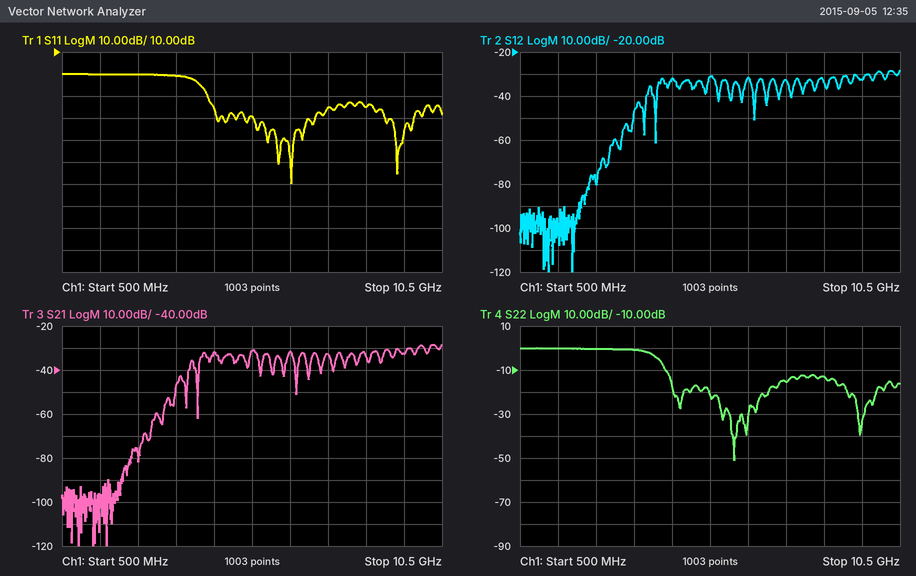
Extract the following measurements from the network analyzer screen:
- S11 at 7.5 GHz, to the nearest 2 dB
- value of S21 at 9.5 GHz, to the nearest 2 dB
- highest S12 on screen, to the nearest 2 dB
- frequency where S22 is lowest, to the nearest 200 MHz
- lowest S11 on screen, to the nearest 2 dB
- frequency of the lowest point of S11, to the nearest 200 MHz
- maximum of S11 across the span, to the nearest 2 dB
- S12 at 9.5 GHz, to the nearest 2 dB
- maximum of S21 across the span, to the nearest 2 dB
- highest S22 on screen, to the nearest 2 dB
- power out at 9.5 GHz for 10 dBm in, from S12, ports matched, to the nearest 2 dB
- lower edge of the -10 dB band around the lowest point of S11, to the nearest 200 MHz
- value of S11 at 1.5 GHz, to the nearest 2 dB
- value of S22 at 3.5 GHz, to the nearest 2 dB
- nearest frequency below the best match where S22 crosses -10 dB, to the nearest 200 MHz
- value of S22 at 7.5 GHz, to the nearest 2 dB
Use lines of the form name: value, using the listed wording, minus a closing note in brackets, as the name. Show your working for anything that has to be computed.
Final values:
S11 at 7.5 GHz, to the nearest 2 dB: -16 dB
value of S21 at 9.5 GHz, to the nearest 2 dB: -32 dB
highest S12 on screen, to the nearest 2 dB: -28 dB
frequency where S22 is lowest, to the nearest 200 MHz: 6.2 GHz
lowest S11 on screen, to the nearest 2 dB: -50 dB
frequency of the lowest point of S11, to the nearest 200 MHz: 6.6 GHz
maximum of S11 across the span, to the nearest 2 dB: 0 dB
S12 at 9.5 GHz, to the nearest 2 dB: -32 dB
maximum of S21 across the span, to the nearest 2 dB: -28 dB
highest S22 on screen, to the nearest 2 dB: 0 dB
power out at 9.5 GHz for 10 dBm in, from S12, ports matched, to the nearest 2 dB: 10 dBm + (-32 dB) = -22 dBm
lower edge of the -10 dB band around the lowest point of S11, to the nearest 200 MHz: 4.4 GHz
value of S11 at 1.5 GHz, to the nearest 2 dB: 0 dB
value of S22 at 3.5 GHz, to the nearest 2 dB: 0 dB
nearest frequency below the best match where S22 crosses -10 dB, to the nearest 200 MHz: 4.4 GHz
value of S22 at 7.5 GHz, to the nearest 2 dB: -16 dB
